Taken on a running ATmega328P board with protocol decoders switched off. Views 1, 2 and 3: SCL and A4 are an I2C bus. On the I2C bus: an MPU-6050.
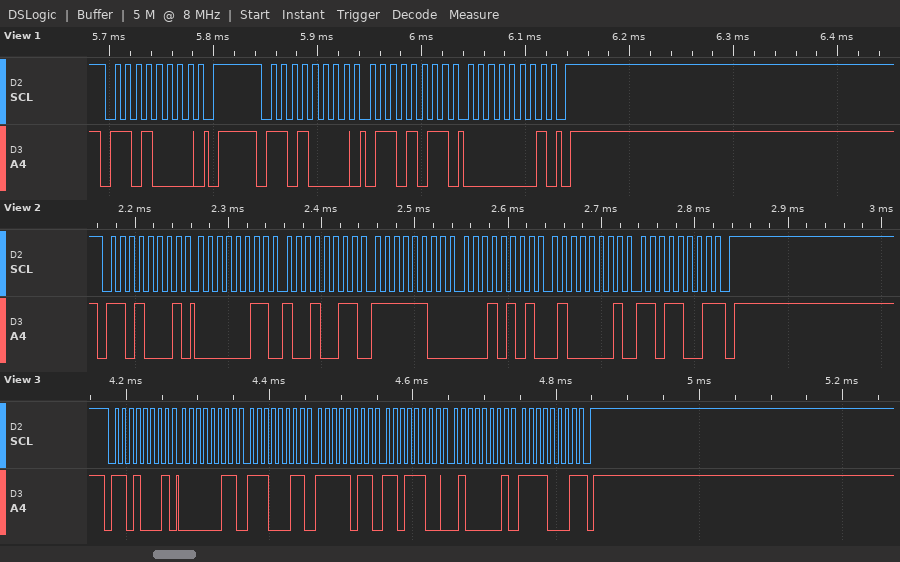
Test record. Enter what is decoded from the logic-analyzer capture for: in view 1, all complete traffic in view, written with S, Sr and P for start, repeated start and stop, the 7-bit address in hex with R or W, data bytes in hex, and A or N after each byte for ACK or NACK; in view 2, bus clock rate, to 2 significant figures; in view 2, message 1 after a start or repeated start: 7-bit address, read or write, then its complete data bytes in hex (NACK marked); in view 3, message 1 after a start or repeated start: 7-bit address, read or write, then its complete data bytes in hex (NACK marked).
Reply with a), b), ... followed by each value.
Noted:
a) S 68W A P S 68W A 6B A 01 A P
b) 100 kHz
c) 0x68 read: 03 93 FC 15 41 D9 NACK
d) 0x68 read: 03 E3 FB DC 41 F1 NACK
